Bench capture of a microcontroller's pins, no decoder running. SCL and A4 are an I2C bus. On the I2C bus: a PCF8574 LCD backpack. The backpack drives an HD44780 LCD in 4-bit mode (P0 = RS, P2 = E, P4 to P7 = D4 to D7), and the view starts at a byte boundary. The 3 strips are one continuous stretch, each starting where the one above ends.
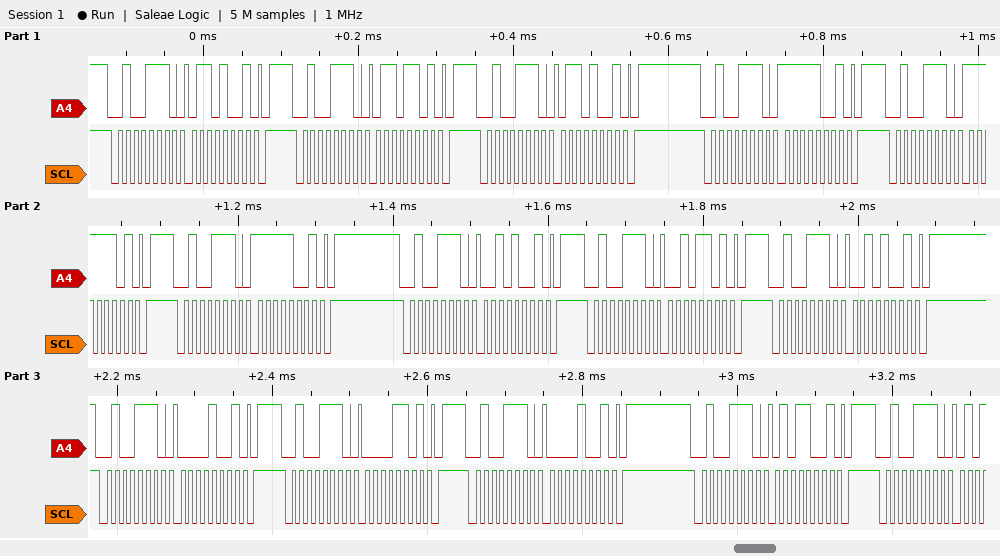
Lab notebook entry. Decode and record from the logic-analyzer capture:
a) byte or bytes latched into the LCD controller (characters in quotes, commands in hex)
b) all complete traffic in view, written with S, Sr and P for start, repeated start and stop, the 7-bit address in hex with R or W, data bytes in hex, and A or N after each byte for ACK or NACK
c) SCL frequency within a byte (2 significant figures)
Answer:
'o' ' '
S 27W A 69 A P S 27W A 6D A P S 27W A 69 A P S 27W A F9 A P S 27W A FD A P S 27W A F9 A P S 27W A 29 A P S 27W A 2D A P S 27W A 29 A P S 27W A 09 A P S 27W A 0D A P S 27W A 09 A P S 27W A 59 A P S 27W A
100 kHz
